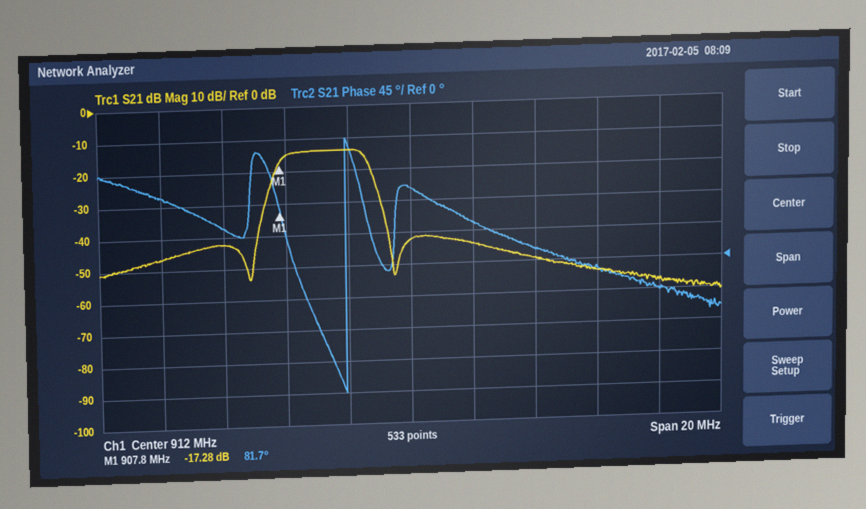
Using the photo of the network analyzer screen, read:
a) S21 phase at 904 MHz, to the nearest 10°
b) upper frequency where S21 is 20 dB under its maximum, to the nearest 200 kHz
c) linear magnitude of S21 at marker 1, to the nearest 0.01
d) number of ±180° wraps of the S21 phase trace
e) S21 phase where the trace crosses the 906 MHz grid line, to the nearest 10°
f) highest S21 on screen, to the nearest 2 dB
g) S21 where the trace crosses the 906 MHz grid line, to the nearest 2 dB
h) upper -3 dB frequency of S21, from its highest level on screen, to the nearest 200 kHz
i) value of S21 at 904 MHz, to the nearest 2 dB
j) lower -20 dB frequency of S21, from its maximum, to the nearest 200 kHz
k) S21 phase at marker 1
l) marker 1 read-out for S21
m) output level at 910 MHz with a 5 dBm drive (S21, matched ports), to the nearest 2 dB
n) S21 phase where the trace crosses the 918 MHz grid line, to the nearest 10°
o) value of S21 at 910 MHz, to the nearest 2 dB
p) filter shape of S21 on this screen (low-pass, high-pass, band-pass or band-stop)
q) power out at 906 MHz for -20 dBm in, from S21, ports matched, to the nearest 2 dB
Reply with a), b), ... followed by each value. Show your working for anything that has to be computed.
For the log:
a) 100°
b) 911.2 MHz
c) 10^(-17.28/20) ≈ 0.14
d) 1
e) 60°
f) -14 dB
g) -42 dB
h) 910.6 MHz
i) -46 dB
j) 907.2 MHz
k) 81.7°
l) -17.28 dB
m) 5 dBm + (-14 dB) = -8 dBm
n) -10°
o) -14 dB
p) band-pass
q) -20 dBm + (-42 dB) = -62 dBm
